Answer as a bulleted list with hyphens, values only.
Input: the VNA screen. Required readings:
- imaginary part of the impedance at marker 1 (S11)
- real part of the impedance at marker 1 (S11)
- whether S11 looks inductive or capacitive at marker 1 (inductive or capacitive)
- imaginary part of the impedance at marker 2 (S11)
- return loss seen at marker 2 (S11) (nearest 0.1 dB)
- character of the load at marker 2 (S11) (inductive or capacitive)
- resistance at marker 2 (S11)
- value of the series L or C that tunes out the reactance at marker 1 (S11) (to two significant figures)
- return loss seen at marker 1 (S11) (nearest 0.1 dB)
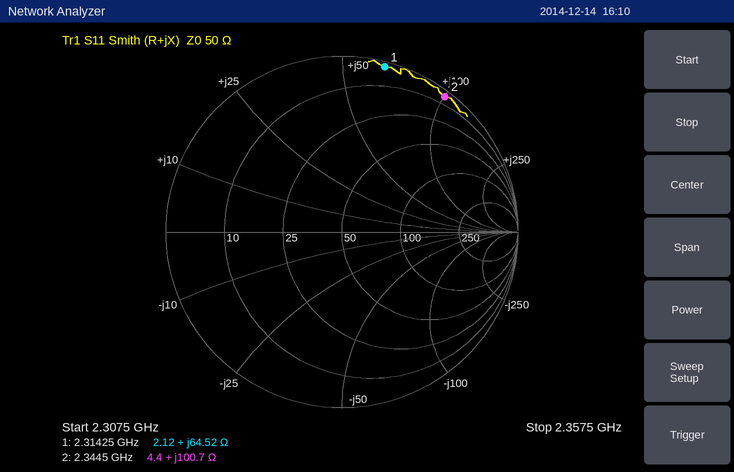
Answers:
- +64.52 Ω
- 2.12 Ω
- inductive
- +100.7 Ω
- 0.3 dB
- inductive
- 4.4 Ω
- 1.1 pF
- 0.3 dB
